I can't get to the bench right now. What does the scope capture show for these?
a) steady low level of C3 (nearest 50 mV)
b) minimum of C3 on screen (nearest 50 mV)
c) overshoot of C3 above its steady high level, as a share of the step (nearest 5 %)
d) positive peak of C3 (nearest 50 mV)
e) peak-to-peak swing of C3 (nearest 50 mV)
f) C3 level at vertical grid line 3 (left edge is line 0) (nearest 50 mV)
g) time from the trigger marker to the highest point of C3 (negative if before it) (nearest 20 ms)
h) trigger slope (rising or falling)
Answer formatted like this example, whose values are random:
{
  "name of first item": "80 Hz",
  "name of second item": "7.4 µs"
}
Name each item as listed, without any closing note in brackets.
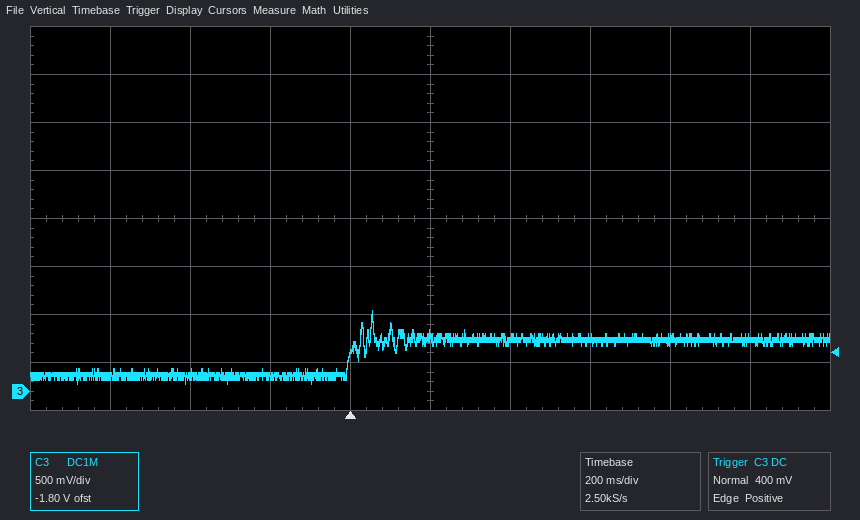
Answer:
{
  "steady low level of C3": "150 mV",
  "minimum of C3 on screen": "100 mV",
  "overshoot of C3 above its steady high level, as a share of the step": "80 %",
  "positive peak of C3": "850 mV",
  "peak-to-peak swing of C3": "750 mV",
  "C3 level at vertical grid line 3 (left edge is line 0)": "150 mV",
  "time from the trigger marker to the highest point of C3 (negative if before it)": "+60 ms",
  "trigger slope": "rising"
}
